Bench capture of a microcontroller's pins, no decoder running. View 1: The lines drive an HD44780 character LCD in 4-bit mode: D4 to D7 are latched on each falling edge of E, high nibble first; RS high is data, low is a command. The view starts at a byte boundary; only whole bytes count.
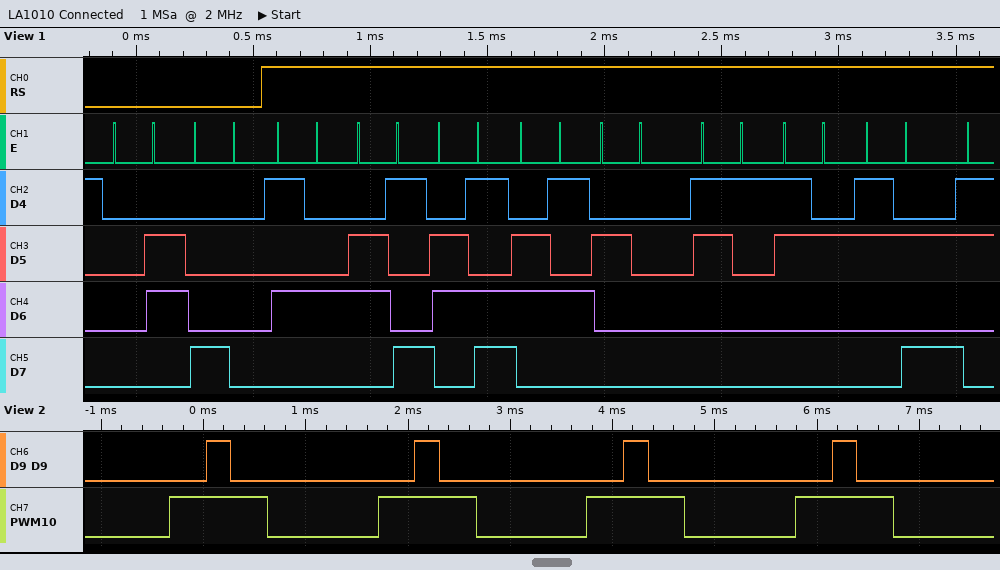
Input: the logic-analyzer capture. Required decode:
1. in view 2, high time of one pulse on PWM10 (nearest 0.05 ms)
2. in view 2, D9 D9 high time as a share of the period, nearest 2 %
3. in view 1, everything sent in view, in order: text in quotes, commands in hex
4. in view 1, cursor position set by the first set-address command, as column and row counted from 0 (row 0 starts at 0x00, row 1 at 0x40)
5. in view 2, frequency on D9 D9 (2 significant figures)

0.95 ms
12 %
0x06 0x80 "Time 12:"
column 0, row 0
490 Hz
